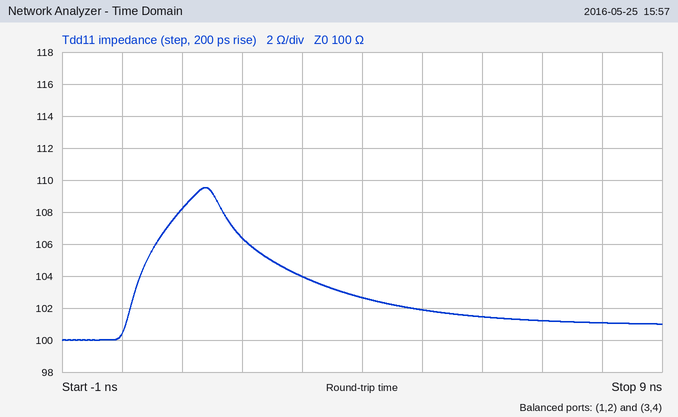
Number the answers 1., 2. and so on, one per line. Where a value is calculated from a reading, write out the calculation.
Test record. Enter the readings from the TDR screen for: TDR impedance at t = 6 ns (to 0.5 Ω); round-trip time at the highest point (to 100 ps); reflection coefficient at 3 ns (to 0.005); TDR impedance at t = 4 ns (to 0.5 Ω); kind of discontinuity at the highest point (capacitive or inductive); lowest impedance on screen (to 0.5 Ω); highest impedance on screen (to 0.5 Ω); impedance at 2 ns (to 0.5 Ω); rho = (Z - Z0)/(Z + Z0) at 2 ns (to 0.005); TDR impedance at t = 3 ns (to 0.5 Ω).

1. 101.5 Ω
2. 1.4 ns
3. (104 − 100)/(104 + 100) ≈ +0.020
4. 102.5 Ω
5. inductive
6. 100.0 Ω
7. 109.5 Ω
8. 106.5 Ω
9. (106.5 − 100)/(106.5 + 100) ≈ +0.0315, so +0.030 to the nearest 0.005
10. 104.0 Ω
